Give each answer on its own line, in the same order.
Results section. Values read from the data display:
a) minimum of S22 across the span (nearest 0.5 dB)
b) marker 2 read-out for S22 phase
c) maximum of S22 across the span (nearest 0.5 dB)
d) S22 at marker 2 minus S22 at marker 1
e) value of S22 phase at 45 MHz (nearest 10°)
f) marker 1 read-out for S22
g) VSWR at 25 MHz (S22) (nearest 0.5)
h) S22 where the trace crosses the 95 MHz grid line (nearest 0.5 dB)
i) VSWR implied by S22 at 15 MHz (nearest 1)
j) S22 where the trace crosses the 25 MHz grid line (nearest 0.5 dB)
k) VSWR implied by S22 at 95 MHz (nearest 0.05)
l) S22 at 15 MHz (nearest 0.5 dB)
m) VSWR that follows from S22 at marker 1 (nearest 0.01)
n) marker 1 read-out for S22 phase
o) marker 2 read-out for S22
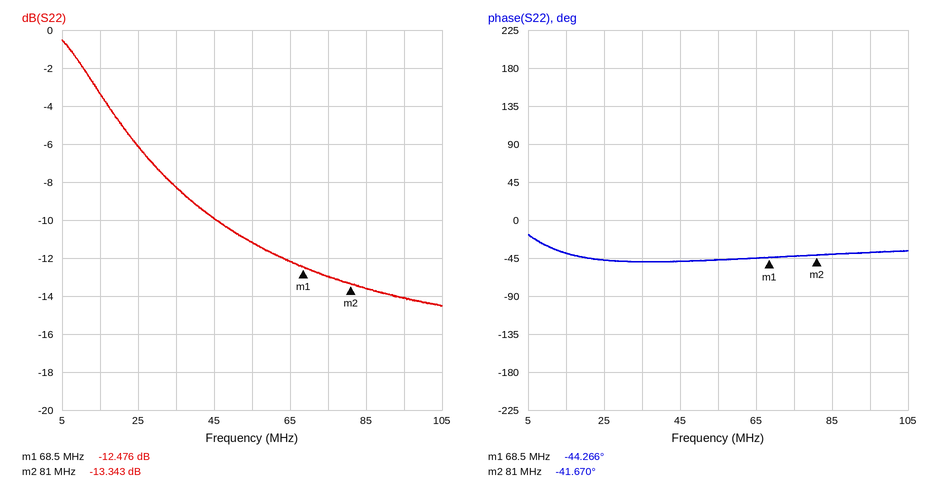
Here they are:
-14.5 dB
-41.670°
-0.5 dB
-0.867 dB
-50°
-12.476 dB
3.0
-14.0 dB
5
-6.0 dB
1.50
-3.5 dB
1.62
-44.266°
-13.343 dB
